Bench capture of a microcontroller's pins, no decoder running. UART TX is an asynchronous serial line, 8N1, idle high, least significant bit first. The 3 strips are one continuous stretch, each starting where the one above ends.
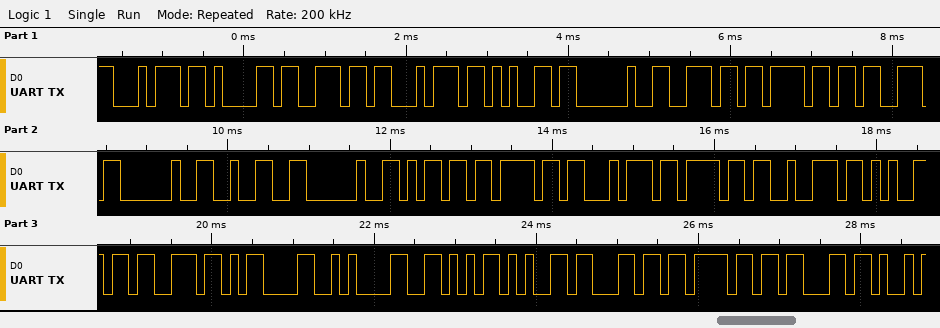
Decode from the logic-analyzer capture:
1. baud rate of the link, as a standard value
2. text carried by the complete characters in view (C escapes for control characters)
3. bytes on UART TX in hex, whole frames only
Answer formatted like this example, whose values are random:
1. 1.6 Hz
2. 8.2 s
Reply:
1. 9600 baud
2. "tante nos 2 motores\r\nVeloc"
3. 74 61 6E 74 65 20 6E 6F 73 20 32 20 6D 6F 74 6F 72 65 73 0D 0A 56 65 6C 6F 63
